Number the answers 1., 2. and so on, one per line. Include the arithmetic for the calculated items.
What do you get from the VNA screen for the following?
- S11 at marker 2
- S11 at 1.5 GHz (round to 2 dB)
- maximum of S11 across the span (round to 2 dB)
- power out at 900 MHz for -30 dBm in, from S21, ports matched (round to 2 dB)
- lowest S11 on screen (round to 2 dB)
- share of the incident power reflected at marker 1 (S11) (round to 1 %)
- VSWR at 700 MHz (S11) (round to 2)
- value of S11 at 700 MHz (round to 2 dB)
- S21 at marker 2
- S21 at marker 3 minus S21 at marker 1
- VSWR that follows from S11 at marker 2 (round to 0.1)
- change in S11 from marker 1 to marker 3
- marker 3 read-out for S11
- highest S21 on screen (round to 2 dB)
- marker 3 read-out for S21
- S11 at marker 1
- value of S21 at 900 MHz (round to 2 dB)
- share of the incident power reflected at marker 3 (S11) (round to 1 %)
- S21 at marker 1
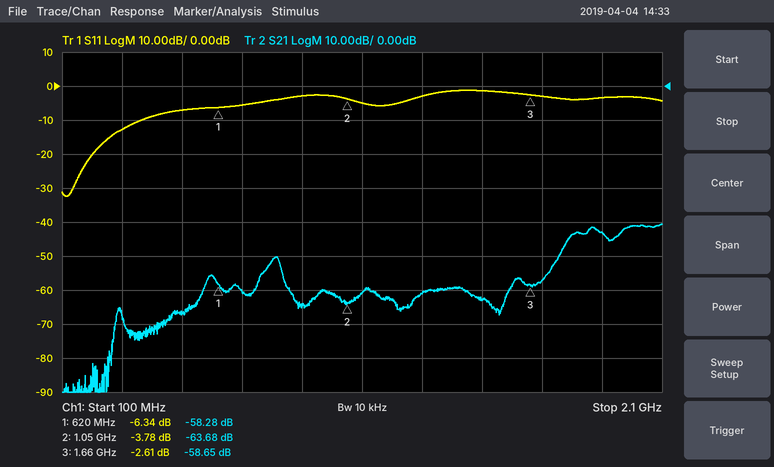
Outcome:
1. -3.78 dB
2. -2 dB
3. -2 dB
4. -30 dBm + (-64 dB) = -94 dBm
5. -32 dB
6. 10^(-6.34/10) ≈ 23 %
7. |Γ| = 10^(-6/20) = 0.5012; VSWR = (1 + 0.5012)/(1 − 0.5012) ≈ 3.01, so 4 to the nearest 2
8. -6 dB
9. -63.68 dB
10. -58.65 − (-58.28) = -0.37 dB
11. (1 + 0.6471)/(1 − 0.6471) ≈ 4.7
12. -2.61 − (-6.34) = 3.73 dB
13. -2.61 dB
14. -40 dB
15. -58.65 dB
16. -6.34 dB
17. -64 dB
18. 10^(-2.61/10) ≈ 55 %
19. -58.28 dB
